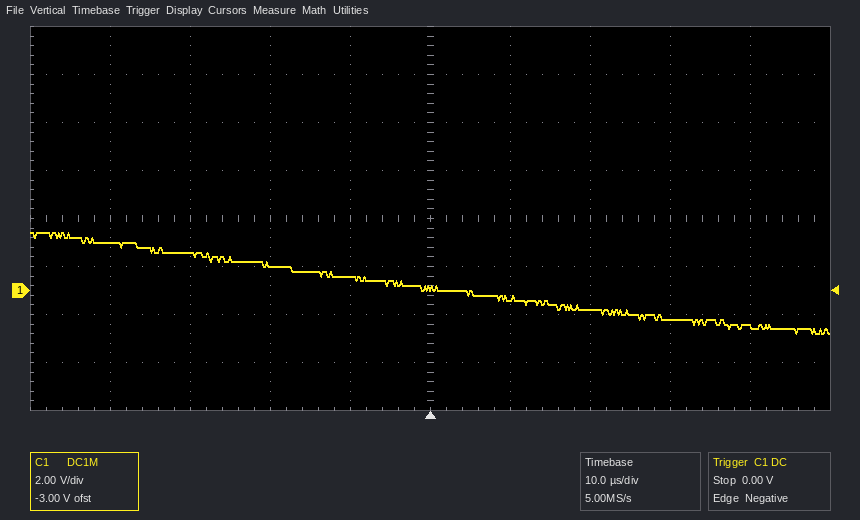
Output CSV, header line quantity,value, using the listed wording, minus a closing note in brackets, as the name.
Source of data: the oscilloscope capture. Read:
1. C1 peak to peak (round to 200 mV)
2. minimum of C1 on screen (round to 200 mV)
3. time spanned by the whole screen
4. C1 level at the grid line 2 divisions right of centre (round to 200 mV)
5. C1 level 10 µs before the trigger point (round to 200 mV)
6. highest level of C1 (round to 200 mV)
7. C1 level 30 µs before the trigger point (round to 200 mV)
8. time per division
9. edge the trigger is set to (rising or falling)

quantity,value
C1 peak to peak,4.2 V
minimum of C1 on screen,-1.8 V
time spanned by the whole screen,100 µs
C1 level at the grid line 2 divisions right of centre,-800 mV
C1 level 10 µs before the trigger point,600 mV
highest level of C1,2.4 V
C1 level 30 µs before the trigger point,1.6 V
time per division,10 µs
edge the trigger is set to,falling
